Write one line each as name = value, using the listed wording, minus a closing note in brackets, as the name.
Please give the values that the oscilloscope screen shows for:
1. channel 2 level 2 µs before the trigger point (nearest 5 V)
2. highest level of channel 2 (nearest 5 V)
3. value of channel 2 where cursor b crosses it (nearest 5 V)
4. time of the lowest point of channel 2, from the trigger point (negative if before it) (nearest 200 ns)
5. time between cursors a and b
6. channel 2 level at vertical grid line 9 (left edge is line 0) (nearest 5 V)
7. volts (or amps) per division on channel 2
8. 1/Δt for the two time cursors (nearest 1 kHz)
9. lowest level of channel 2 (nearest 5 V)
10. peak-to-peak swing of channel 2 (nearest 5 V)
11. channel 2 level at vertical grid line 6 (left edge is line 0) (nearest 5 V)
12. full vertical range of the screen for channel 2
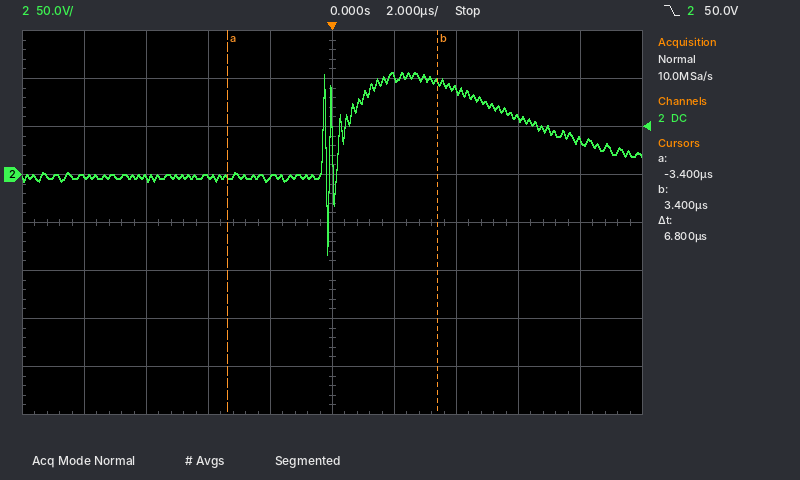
channel 2 level 2 µs before the trigger point = -5 V
highest level of channel 2 = 105 V
value of channel 2 where cursor b crosses it = 95 V
time of the lowest point of channel 2, from the trigger point (negative if before it) = -200 ns
time between cursors a and b = 6.8 µs
channel 2 level at vertical grid line 9 (left edge is line 0) = 35 V
volts (or amps) per division on channel 2 = 50 V
1/Δt for the two time cursors = 147 kHz
lowest level of channel 2 = -85 V
peak-to-peak swing of channel 2 = 190 V
channel 2 level at vertical grid line 6 (left edge is line 0) = 100 V
full vertical range of the screen for channel 2 = 400 V
